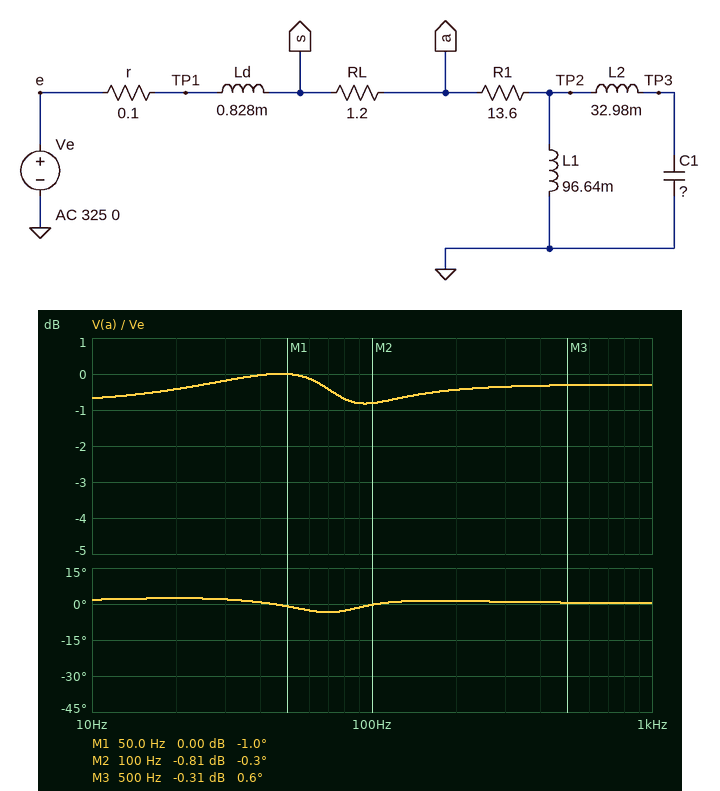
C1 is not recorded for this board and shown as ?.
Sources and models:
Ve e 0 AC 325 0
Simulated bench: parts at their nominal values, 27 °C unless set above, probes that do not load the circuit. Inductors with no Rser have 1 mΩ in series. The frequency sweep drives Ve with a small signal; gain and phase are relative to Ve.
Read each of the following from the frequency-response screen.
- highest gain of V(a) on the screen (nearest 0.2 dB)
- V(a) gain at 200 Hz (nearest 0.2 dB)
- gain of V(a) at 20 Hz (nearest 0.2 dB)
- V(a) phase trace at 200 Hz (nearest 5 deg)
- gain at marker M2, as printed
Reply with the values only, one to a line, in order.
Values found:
0 dB
-0.4 dB
-0.4 dB
0 deg
-0.81 dB
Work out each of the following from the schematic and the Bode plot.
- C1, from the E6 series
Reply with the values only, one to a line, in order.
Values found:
100 µF
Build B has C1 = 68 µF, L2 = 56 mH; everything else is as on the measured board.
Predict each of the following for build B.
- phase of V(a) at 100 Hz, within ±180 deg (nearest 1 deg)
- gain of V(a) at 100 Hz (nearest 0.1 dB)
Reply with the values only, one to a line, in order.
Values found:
1 deg
-0.7 dB
